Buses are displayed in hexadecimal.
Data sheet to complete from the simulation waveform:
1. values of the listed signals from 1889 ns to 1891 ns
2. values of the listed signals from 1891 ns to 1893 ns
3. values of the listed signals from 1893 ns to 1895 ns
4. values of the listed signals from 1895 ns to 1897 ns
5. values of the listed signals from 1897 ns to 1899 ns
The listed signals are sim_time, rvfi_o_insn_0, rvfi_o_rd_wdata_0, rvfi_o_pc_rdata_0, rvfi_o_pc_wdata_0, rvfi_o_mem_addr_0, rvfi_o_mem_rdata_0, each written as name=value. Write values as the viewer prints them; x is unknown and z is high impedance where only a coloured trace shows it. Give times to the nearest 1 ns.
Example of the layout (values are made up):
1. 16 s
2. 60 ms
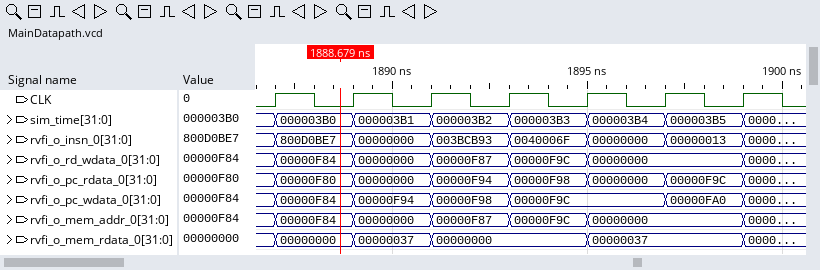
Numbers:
1. sim_time=000003B1, rvfi_o_insn_0=00000000, rvfi_o_rd_wdata_0=00000000, rvfi_o_pc_rdata_0=00000000, rvfi_o_pc_wdata_0=00000F94, rvfi_o_mem_addr_0=00000000, rvfi_o_mem_rdata_0=00000037
2. sim_time=000003B2, rvfi_o_insn_0=003BCB93, rvfi_o_rd_wdata_0=00000F87, rvfi_o_pc_rdata_0=00000F94, rvfi_o_pc_wdata_0=00000F98, rvfi_o_mem_addr_0=00000F87, rvfi_o_mem_rdata_0=00000000
3. sim_time=000003B3, rvfi_o_insn_0=0040006F, rvfi_o_rd_wdata_0=00000F9C, rvfi_o_pc_rdata_0=00000F98, rvfi_o_pc_wdata_0=00000F9C, rvfi_o_mem_addr_0=00000F9C, rvfi_o_mem_rdata_0=00000000
4. sim_time=000003B4, rvfi_o_insn_0=00000000, rvfi_o_rd_wdata_0=00000000, rvfi_o_pc_rdata_0=00000000, rvfi_o_pc_wdata_0=00000F9C, rvfi_o_mem_addr_0=00000000, rvfi_o_mem_rdata_0=00000037
5. sim_time=000003B5, rvfi_o_insn_0=00000013, rvfi_o_rd_wdata_0=00000000, rvfi_o_pc_rdata_0=00000F9C, rvfi_o_pc_wdata_0=00000FA0, rvfi_o_mem_addr_0=00000000, rvfi_o_mem_rdata_0=00000037
